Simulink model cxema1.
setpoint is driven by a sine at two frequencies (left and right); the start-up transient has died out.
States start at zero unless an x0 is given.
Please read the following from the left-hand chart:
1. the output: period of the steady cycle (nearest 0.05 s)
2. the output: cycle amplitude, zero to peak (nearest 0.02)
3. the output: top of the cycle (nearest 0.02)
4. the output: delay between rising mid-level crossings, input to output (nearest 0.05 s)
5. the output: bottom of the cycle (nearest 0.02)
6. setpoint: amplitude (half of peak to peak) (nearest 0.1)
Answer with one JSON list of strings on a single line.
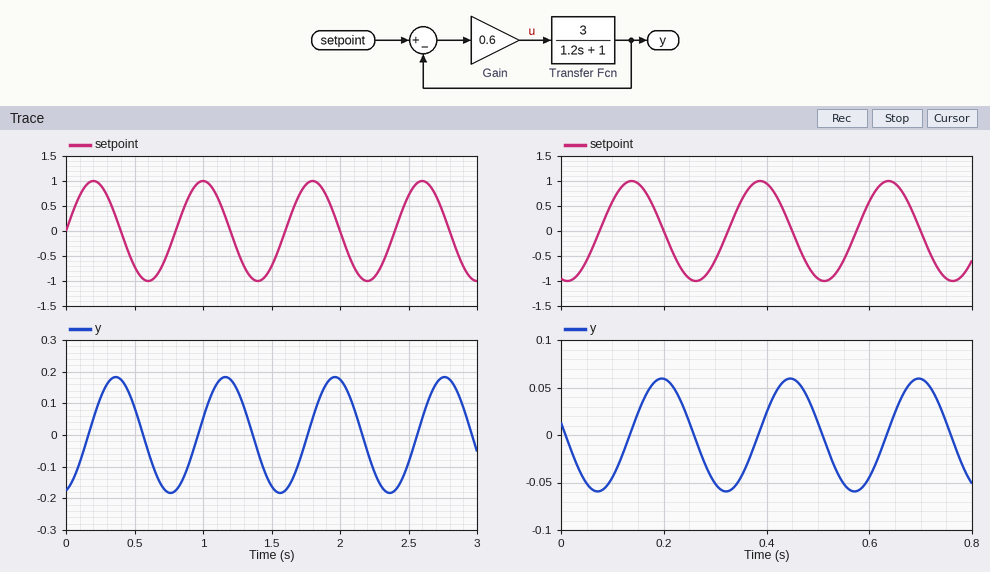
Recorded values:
["0.80 s", "0.18", "0.18", "0.15 s", "-0.18", "1.0"]
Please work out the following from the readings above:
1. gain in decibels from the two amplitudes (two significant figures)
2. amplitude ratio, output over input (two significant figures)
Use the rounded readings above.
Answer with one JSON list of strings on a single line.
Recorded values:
["-15 dB", "0.18"]
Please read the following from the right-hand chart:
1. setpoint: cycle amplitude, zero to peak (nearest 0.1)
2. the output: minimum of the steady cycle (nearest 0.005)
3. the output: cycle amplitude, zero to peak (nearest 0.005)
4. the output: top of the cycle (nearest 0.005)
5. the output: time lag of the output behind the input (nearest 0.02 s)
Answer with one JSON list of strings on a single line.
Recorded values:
["1.0", "-0.060", "0.060", "0.060", "0.06 s"]
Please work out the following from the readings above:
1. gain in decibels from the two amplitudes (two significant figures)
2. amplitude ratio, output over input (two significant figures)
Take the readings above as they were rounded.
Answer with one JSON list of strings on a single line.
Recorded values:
["-24 dB", "0.060"]
